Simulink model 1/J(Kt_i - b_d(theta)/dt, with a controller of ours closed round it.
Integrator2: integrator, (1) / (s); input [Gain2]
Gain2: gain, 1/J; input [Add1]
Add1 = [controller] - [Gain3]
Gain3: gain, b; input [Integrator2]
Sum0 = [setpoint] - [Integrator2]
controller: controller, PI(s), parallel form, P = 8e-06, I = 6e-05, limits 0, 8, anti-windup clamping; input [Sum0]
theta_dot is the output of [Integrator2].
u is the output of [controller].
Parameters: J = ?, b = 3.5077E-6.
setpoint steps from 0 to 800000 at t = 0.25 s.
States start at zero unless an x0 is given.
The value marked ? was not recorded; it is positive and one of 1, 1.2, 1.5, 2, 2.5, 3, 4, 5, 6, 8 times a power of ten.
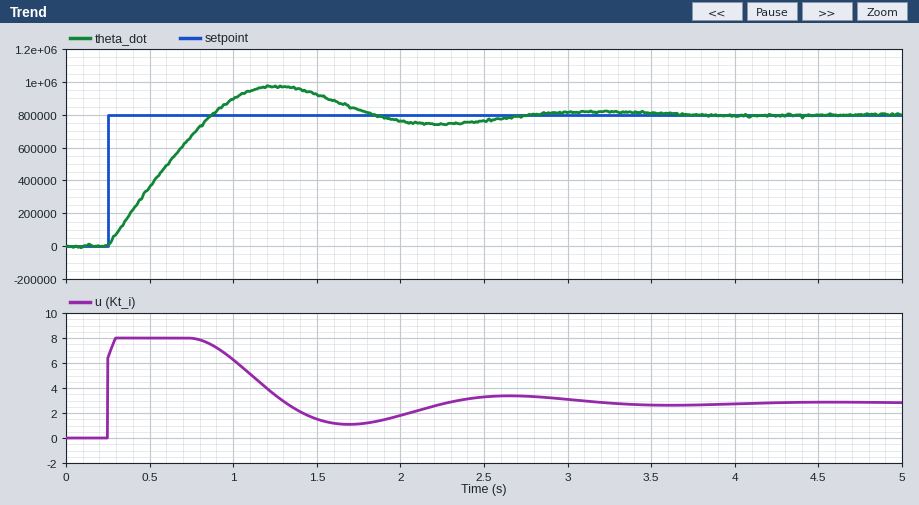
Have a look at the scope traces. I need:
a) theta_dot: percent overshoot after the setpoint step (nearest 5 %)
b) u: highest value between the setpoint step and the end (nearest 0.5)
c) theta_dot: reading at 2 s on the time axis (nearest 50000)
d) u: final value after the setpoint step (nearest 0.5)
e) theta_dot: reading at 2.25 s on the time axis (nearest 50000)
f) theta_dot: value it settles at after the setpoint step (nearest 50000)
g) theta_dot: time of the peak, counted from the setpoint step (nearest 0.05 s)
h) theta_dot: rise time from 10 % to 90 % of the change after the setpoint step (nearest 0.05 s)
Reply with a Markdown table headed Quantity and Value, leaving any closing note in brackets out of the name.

| Quantity | Value |
|---|---|
| theta_dot: percent overshoot after the setpoint step | 20 % |
| u: highest value between the setpoint step and the end | 8.0 |
| theta_dot: reading at 2 s on the time axis | 750000 |
| u: final value after the setpoint step | 3.0 |
| theta_dot: reading at 2.25 s on the time axis | 750000 |
| theta_dot: value it settles at after the setpoint step | 800000 |
| theta_dot: time of the peak, counted from the setpoint step | 1.00 s |
| theta_dot: rise time from 10 % to 90 % of the change after the setpoint step | 0.50 s |
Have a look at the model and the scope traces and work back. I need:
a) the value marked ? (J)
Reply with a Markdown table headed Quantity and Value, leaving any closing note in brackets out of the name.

| Quantity | Value |
|---|---|
| the value marked ? | 5e-06 |
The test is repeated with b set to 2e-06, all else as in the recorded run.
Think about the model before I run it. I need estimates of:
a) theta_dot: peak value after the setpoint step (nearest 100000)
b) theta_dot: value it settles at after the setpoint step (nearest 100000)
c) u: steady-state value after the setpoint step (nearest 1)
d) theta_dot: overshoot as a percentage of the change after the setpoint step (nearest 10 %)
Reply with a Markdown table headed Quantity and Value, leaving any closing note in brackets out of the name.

| Quantity | Value |
|---|---|
| theta_dot: peak value after the setpoint step | 1000000 |
| theta_dot: value it settles at after the setpoint step | 800000 |
| u: steady-state value after the setpoint step | 2 |
| theta_dot: overshoot as a percentage of the change after the setpoint step | 30 % |
